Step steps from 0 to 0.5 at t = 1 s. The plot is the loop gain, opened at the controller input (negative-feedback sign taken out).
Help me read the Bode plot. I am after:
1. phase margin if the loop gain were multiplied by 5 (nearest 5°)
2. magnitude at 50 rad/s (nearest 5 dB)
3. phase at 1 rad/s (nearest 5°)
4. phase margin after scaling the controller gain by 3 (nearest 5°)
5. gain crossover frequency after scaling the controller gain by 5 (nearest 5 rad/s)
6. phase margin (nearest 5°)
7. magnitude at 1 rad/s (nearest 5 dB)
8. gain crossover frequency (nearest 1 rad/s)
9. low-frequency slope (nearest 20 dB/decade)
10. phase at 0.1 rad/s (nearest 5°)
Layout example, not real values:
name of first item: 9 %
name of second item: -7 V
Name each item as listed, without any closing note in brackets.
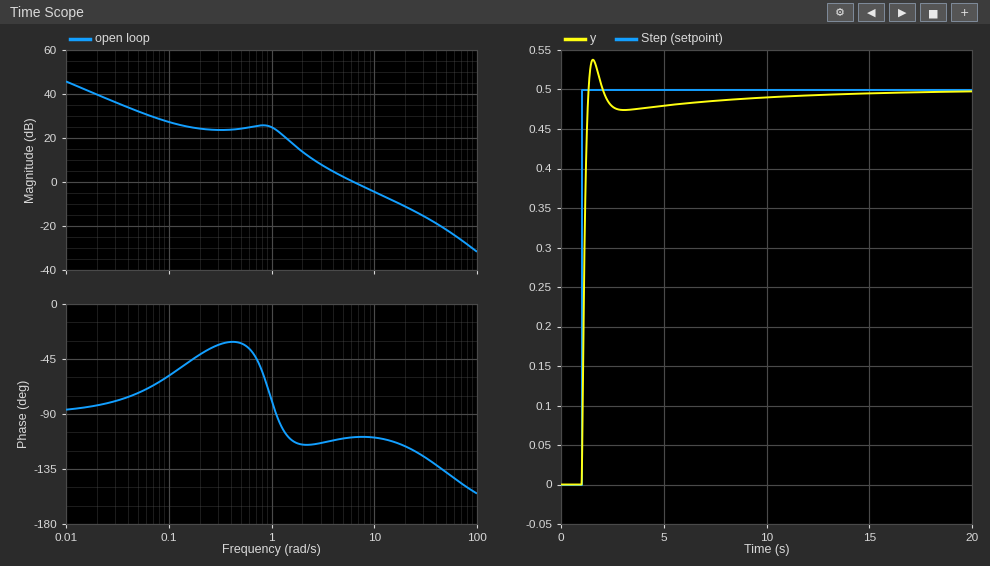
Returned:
phase margin if the loop gain were multiplied by 5: 60°
magnitude at 50 rad/s: -20 dB
phase at 1 rad/s: -80°
phase margin after scaling the controller gain by 3: 65°
gain crossover frequency after scaling the controller gain by 5: 25 rad/s
phase margin: 70°
magnitude at 1 rad/s: 25 dB
gain crossover frequency: 6 rad/s
low-frequency slope: -20 dB/decade
phase at 0.1 rad/s: -60°
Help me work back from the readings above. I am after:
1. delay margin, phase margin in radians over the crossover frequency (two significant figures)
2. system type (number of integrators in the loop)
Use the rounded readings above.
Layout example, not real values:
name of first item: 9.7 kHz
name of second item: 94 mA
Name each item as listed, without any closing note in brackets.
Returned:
delay margin, phase margin in radians over the crossover frequency: 0.20 s
system type: 1
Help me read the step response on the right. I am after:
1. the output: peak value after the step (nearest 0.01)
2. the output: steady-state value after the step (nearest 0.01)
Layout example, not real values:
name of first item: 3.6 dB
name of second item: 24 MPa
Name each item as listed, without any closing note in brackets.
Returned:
the output: peak value after the step: 0.54
the output: steady-state value after the step: 0.50
